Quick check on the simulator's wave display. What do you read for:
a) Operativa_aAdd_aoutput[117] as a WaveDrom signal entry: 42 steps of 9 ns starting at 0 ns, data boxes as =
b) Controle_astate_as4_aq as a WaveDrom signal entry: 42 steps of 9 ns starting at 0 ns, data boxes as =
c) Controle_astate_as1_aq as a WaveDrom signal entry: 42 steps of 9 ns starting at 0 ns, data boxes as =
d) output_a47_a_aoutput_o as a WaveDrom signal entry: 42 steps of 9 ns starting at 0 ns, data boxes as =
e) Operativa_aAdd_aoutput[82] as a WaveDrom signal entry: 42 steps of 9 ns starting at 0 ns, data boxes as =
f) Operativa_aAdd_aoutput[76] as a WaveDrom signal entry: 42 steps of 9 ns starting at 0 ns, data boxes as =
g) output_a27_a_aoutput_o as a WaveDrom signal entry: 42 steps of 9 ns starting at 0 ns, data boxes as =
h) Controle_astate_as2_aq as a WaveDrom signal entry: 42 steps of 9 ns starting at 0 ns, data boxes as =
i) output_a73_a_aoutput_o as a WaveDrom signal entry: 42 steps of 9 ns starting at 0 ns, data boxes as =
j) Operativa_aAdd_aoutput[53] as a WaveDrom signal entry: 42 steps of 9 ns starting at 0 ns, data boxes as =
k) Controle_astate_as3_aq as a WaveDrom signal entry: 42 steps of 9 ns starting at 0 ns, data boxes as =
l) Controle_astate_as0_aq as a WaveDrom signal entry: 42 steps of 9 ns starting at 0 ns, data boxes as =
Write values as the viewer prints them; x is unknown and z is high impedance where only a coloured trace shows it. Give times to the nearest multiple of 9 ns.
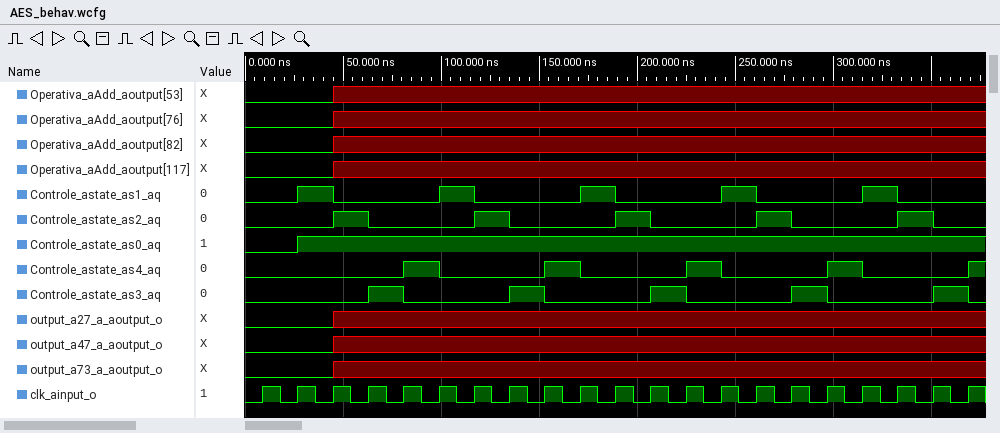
{name: 'Operativa_aAdd_aoutput[117]', wave: '0....x....................................'}
{name: 'Controle_astate_as4_aq', wave: '0........1.0.....1.0.....1.0.....1.0.....1'}
{name: 'Controle_astate_as1_aq', wave: '0..1.0.....1.0.....1.0.....1.0.....1.0....'}
{name: 'output_a47_a_aoutput_o', wave: '0....x....................................'}
{name: 'Operativa_aAdd_aoutput[82]', wave: '0....x....................................'}
{name: 'Operativa_aAdd_aoutput[76]', wave: '0....x....................................'}
{name: 'output_a27_a_aoutput_o', wave: '0....x....................................'}
{name: 'Controle_astate_as2_aq', wave: '0....1.0.....1.0.....1.0.....1.0.....1.0..'}
{name: 'output_a73_a_aoutput_o', wave: '0....x....................................'}
{name: 'Operativa_aAdd_aoutput[53]', wave: '0....x....................................'}
{name: 'Controle_astate_as3_aq', wave: '0......1.0.....1.0.....1.0.....1.0.....1.0'}
{name: 'Controle_astate_as0_aq', wave: '0..1......................................'}
